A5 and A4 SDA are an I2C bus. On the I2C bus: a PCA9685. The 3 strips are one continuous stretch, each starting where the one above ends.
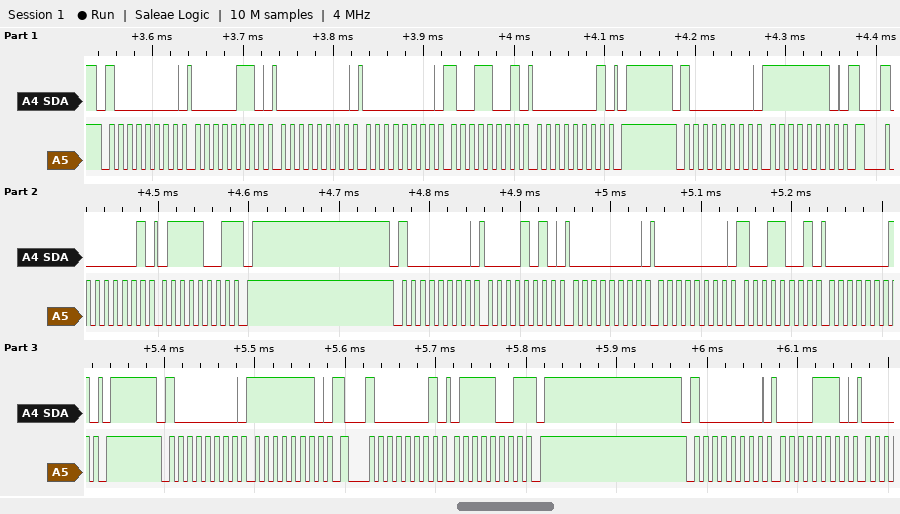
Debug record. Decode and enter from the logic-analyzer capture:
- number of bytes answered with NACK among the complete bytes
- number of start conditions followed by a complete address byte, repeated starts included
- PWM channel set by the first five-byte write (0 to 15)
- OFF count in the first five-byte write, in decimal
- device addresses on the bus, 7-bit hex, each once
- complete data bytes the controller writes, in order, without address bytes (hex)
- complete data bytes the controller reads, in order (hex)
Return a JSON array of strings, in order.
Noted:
["2", "7", "0", "409", "0x40", "06 00 00 99 01 FE 0A 00 00 99 01 FE 0E", "79 79"]
